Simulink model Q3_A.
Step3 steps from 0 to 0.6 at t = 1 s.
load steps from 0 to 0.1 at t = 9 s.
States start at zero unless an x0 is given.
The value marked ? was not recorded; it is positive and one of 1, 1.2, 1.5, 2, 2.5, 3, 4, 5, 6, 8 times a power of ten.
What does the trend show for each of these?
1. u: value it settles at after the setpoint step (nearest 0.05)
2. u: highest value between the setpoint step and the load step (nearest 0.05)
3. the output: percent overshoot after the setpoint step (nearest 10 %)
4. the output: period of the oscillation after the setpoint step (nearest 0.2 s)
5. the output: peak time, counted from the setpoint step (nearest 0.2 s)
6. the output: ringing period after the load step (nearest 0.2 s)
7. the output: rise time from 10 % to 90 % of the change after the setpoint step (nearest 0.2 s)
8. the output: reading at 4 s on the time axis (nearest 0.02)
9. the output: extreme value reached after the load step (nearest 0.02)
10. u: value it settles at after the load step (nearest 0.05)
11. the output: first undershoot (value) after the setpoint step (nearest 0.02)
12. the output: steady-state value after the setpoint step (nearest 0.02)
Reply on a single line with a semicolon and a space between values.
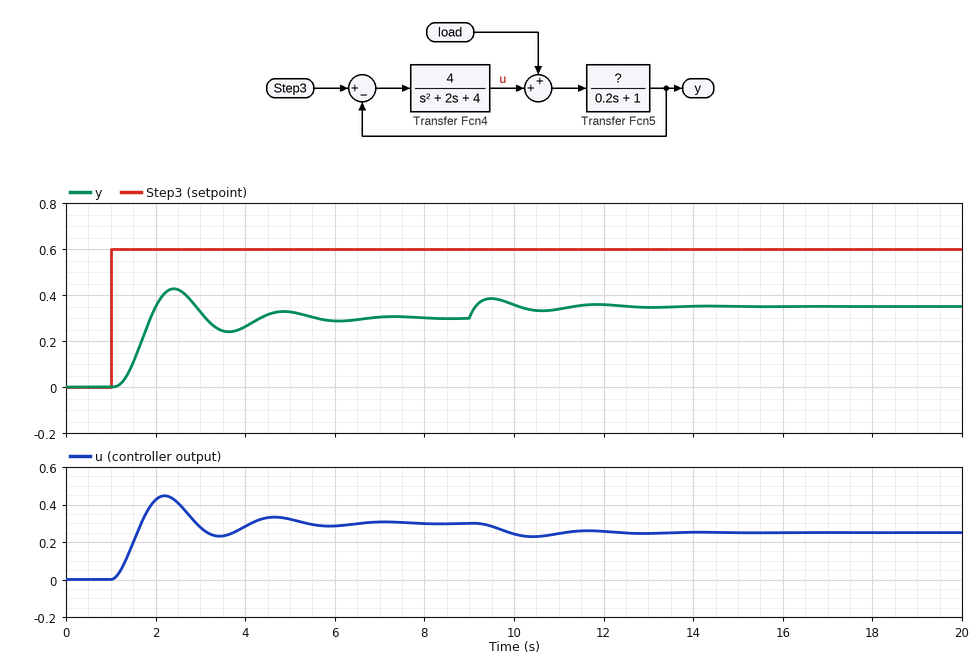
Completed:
0.30; 0.45; 40 %; 2.4 s; 1.4 s; 2.4 s; 0.6 s; 0.26; 0.38; 0.25; 0.24; 0.30
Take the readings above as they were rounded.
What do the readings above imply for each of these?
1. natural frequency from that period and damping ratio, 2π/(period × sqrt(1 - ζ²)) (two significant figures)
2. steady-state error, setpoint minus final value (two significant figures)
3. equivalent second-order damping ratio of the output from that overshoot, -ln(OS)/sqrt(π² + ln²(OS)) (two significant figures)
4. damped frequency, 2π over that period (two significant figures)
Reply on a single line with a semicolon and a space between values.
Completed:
2.7 rad/s; 0.30; 0.28; 2.6 rad/s
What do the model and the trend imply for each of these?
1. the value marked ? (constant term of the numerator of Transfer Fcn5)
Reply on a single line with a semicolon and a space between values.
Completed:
1
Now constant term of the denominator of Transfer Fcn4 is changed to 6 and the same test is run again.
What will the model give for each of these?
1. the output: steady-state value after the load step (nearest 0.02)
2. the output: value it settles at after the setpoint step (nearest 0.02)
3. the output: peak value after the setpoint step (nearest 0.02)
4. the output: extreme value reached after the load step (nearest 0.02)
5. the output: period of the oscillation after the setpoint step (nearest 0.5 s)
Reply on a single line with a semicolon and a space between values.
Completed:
0.30; 0.24; 0.34; 0.32; 2.0 s
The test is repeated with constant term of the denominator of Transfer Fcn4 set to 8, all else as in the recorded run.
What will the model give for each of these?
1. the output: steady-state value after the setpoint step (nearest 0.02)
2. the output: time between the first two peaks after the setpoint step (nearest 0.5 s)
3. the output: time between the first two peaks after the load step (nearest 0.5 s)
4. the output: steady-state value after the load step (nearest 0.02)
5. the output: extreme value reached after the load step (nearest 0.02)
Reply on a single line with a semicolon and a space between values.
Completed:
0.20; 2.0 s; 2.0 s; 0.26; 0.28
